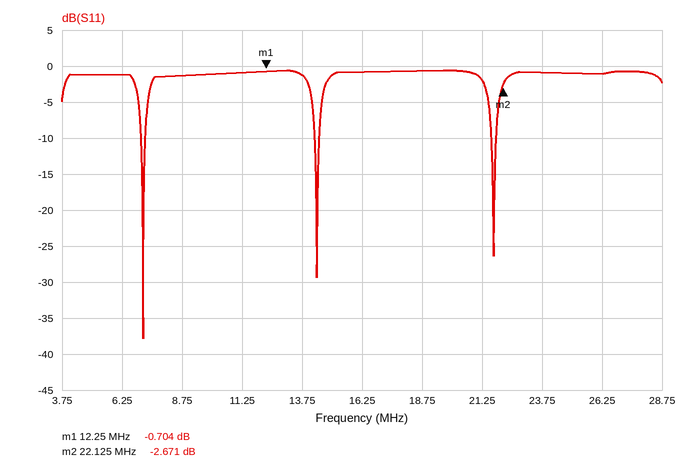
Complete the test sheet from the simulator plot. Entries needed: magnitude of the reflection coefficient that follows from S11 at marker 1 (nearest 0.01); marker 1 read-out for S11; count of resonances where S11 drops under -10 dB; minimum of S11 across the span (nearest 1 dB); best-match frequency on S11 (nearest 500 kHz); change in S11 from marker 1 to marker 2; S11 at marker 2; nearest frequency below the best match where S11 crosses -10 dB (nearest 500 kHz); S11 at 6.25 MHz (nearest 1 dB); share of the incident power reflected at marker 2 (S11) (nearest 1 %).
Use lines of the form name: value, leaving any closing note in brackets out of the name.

magnitude of the reflection coefficient that follows from S11 at marker 1: 0.92
marker 1 read-out for S11: -0.704 dB
count of resonances where S11 drops under -10 dB: 3
minimum of S11 across the span: -38 dB
best-match frequency on S11: 7.0 MHz
change in S11 from marker 1 to marker 2: -1.967 dB
S11 at marker 2: -2.671 dB
nearest frequency below the best match where S11 crosses -10 dB: 7.0 MHz
S11 at 6.25 MHz: -1 dB
share of the incident power reflected at marker 2 (S11): 54 %
